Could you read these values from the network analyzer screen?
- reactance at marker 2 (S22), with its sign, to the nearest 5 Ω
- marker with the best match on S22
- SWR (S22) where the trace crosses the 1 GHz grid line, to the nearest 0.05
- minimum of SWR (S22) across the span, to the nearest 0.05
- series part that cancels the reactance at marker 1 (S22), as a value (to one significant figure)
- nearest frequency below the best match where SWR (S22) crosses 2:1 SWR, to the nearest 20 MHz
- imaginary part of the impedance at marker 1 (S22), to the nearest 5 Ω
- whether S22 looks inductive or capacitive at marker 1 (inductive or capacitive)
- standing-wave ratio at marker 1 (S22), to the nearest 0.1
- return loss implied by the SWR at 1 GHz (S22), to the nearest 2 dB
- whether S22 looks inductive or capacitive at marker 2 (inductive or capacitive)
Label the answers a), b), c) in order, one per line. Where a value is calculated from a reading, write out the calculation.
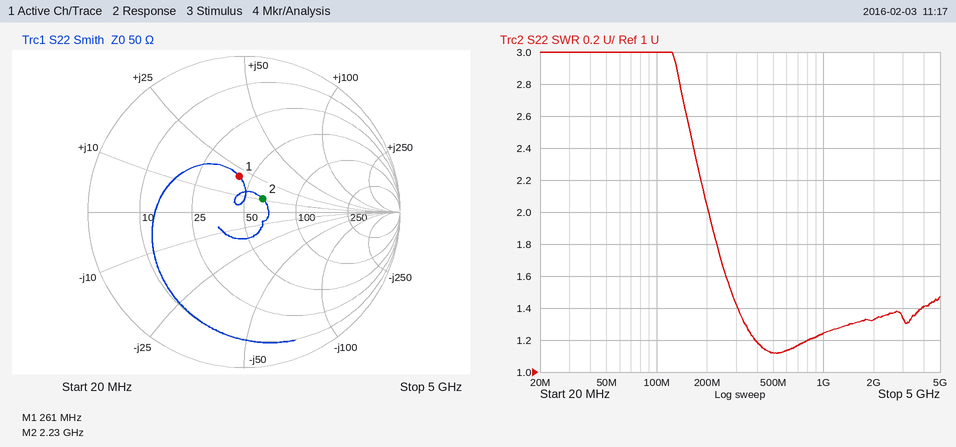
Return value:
a) +10 Ω
b) marker 2
c) 1.25
d) 1.10
e) C = 1/(2π × 261 MHz × 20 Ω) ≈ 30 pF
f) 200 MHz
g) +20 Ω
h) inductive
i) 1.6
j) −20 log10((1.25 − 1)/(1.25 + 1)) ≈ 19.1 dB, so 20 dB to the nearest 2 dB
k) inductive
